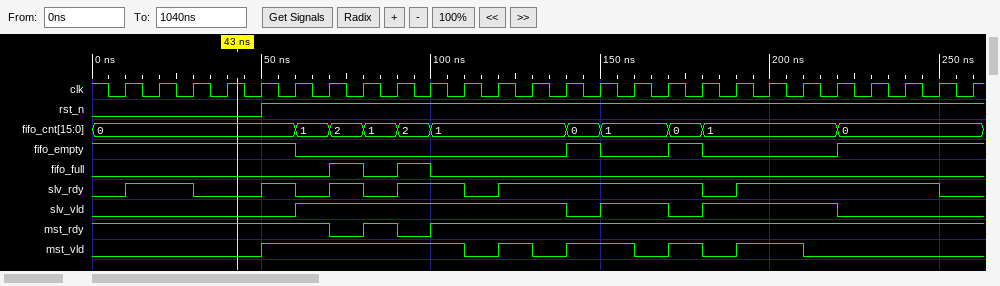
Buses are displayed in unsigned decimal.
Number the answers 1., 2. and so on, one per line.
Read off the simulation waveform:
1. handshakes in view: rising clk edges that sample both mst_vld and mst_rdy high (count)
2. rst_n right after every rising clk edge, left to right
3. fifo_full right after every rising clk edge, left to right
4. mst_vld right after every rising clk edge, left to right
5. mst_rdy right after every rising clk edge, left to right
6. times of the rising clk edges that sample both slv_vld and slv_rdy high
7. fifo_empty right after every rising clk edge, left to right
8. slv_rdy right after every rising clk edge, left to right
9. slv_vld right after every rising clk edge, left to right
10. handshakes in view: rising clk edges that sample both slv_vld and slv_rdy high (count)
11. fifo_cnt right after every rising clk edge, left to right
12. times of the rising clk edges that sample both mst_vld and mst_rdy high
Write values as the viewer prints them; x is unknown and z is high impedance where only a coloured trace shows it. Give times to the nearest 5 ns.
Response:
1. 10
2. 0 0 0 0 1 1 1 1 1 1 1 1 1 1 1 1 1 1 1 1 1 1 1 1 1 1
3. 0 0 0 0 0 0 1 0 1 0 0 0 0 0 0 0 0 0 0 0 0 0 0 0 0 0
4. 0 0 0 0 1 1 1 1 1 1 0 1 0 1 1 0 1 0 1 1 0 0 0 0 0 0
5. 1 1 1 1 1 1 0 1 0 1 1 1 1 1 1 1 1 1 1 1 1 1 1 1 1 1
6. 80 ns, 100 ns, 110 ns, 130 ns, 140 ns, 160 ns, 170 ns, 200 ns, 210 ns, 220 ns
7. 1 1 1 1 1 0 0 0 0 0 0 0 0 1 0 0 1 0 0 0 0 1 1 1 1 1
8. 1 1 0 0 1 0 1 0 1 1 0 1 1 1 1 1 1 0 1 1 1 1 1 1 0 0
9. 0 0 0 0 0 1 1 1 1 1 1 1 1 0 1 1 0 1 1 1 1 0 0 0 0 0
10. 10
11. 0, 0, 0, 0, 0, 1, 2, 1, 2, 1, 1, 1, 1, 0, 1, 1, 0, 1, 1, 1, 1, 0, 0, 0, 0, 0
12. 60 ns, 70 ns, 90 ns, 110 ns, 130 ns, 150 ns, 160 ns, 180 ns, 200 ns, 210 ns
